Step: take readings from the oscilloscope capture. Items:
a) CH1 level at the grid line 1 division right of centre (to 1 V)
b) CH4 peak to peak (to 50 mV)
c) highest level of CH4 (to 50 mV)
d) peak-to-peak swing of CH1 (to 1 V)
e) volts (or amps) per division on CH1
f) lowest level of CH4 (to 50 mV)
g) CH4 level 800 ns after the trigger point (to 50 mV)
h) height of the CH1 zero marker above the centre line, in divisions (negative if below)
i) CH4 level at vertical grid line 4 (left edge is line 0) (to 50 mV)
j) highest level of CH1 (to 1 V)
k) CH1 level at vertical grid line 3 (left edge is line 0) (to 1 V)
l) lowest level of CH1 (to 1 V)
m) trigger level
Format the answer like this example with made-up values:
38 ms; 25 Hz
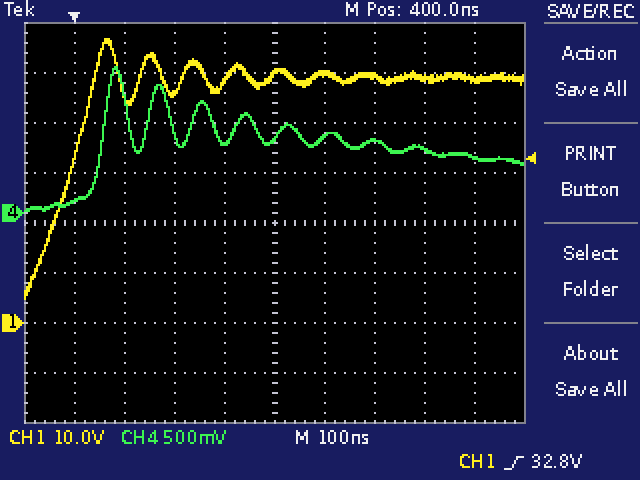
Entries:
50 V; 1.45 V; 1.45 V; 52 V; 10 V; 0 mV; 550 mV; -2.0 div; 700 mV; 57 V; 46 V; 5 V; 32.8 V
